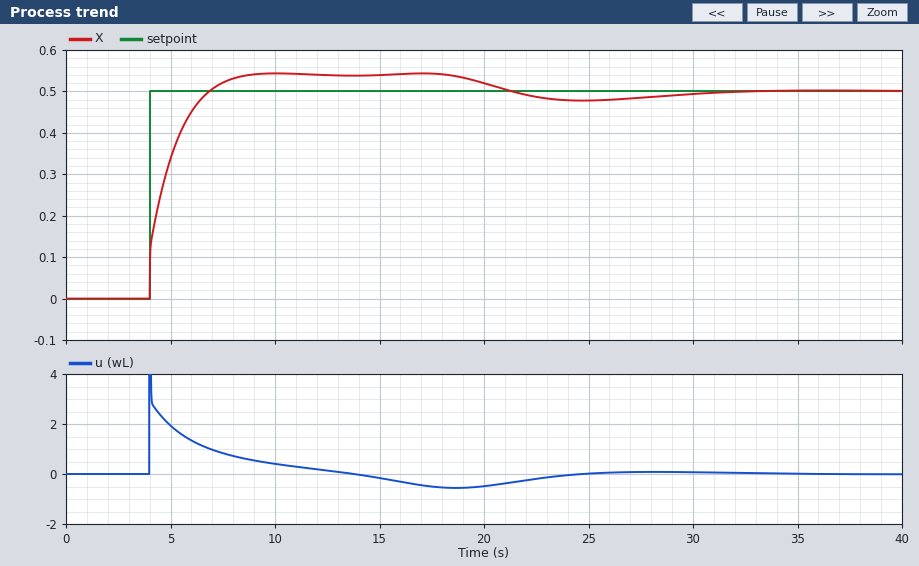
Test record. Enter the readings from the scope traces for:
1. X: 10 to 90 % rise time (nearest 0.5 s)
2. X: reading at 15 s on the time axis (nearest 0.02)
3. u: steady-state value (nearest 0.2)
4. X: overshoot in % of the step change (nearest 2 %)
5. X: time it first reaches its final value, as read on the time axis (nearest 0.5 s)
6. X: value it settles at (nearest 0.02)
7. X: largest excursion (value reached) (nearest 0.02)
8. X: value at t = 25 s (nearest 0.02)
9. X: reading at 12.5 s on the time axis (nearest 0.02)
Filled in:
2.0 s
0.54
0.0
8 %
7.0 s
0.50
0.54
0.48
0.54
